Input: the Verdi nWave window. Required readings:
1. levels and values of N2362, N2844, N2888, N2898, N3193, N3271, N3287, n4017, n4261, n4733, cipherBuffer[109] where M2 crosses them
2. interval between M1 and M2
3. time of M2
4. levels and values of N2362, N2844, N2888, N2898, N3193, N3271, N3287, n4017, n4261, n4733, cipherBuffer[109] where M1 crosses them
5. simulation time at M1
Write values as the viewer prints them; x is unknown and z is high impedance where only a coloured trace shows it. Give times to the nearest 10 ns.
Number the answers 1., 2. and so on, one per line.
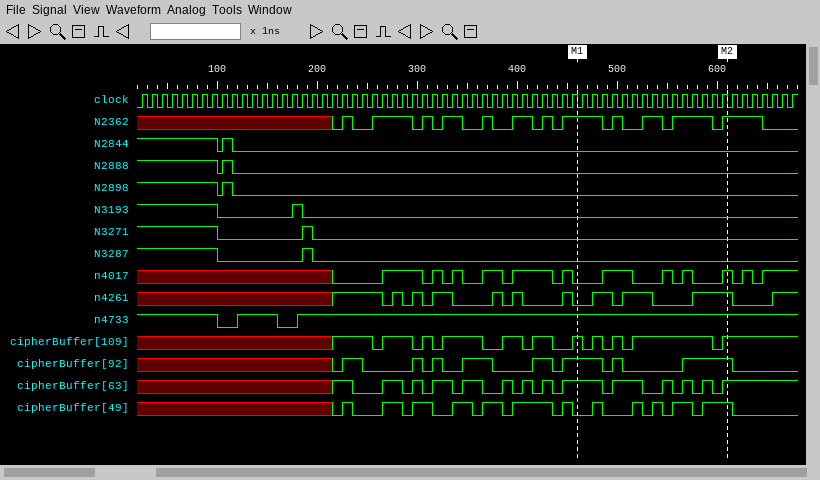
1. N2362=1, N2844=0, N2888=0, N2898=0, N3193=0, N3271=0, N3287=0, n4017=1, n4261=1, n4733=1, cipherBuffer[109]=1
2. 150 ns
3. 610 ns
4. N2362=1, N2844=0, N2888=0, N2898=0, N3193=0, N3271=0, N3287=0, n4017=0, n4261=0, n4733=1, cipherBuffer[109]=1
5. 460 ns
